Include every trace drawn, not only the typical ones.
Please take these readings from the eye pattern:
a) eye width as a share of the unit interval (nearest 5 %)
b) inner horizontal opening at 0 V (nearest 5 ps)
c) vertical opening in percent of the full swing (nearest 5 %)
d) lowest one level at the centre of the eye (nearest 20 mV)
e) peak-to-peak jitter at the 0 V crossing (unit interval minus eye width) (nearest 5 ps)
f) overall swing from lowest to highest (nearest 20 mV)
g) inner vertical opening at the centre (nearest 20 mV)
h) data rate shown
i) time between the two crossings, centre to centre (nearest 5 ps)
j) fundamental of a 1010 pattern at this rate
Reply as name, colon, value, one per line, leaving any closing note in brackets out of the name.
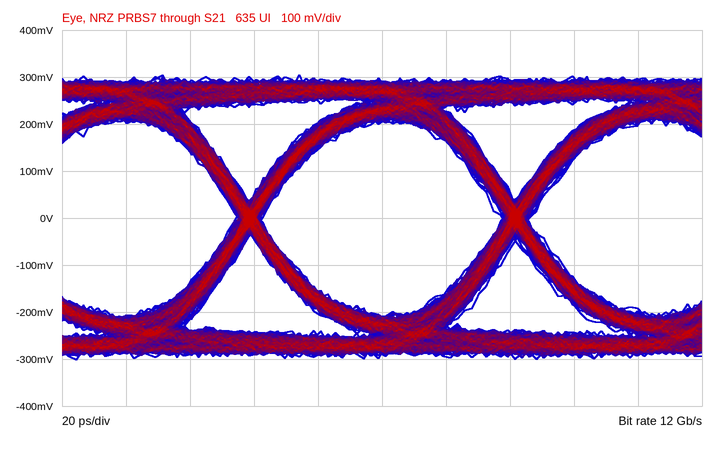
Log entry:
eye width as a share of the unit interval: 90 %
inner horizontal opening at 0 V: 75 ps
vertical opening in percent of the full swing: 70 %
lowest one level at the centre of the eye: 200 mV
peak-to-peak jitter at the 0 V crossing (unit interval minus eye width): 10 ps
overall swing from lowest to highest: 600 mV
inner vertical opening at the centre: 420 mV
data rate shown: 12 Gb/s
time between the two crossings, centre to centre: 85 ps
fundamental of a 1010 pattern at this rate: 6 GHz
